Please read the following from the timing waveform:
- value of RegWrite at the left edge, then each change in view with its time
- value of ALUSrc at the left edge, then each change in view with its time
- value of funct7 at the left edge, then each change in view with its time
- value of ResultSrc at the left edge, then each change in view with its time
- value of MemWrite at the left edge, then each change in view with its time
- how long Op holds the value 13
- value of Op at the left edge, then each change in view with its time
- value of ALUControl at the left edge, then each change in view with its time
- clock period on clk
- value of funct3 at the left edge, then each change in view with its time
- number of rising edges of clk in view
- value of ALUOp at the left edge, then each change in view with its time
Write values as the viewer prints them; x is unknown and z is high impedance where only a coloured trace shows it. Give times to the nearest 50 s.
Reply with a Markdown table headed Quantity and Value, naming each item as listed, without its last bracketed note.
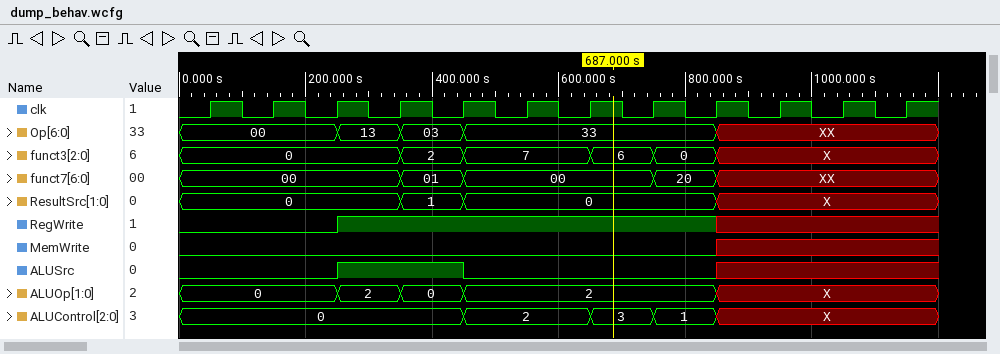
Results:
| Quantity | Value |
|---|---|
| value of RegWrite at the left edge, then each change in view with its time | 0, 1 at 250 s, x at 850 s |
| value of ALUSrc at the left edge, then each change in view with its time | 0, 1 at 250 s, 0 at 450 s, x at 850 s |
| value of funct7 at the left edge, then each change in view with its time | 00, 01 at 350 s, 00 at 450 s, 20 at 750 s, XX at 850 s |
| value of ResultSrc at the left edge, then each change in view with its time | 0, 1 at 350 s, 0 at 450 s, X at 850 s |
| value of MemWrite at the left edge, then each change in view with its time | 0, x at 850 s |
| how long Op holds the value 13 | 100 s |
| value of Op at the left edge, then each change in view with its time | 00, 13 at 250 s, 03 at 350 s, 33 at 450 s, XX at 850 s |
| value of ALUControl at the left edge, then each change in view with its time | 0, 2 at 450 s, 3 at 650 s, 1 at 750 s, X at 850 s |
| clock period on clk | 100 s |
| value of funct3 at the left edge, then each change in view with its time | 0, 2 at 350 s, 7 at 450 s, 6 at 650 s, 0 at 750 s, X at 850 s |
| number of rising edges of clk in view | 12 |
| value of ALUOp at the left edge, then each change in view with its time | 0, 2 at 250 s, 0 at 350 s, 2 at 450 s, X at 850 s |
